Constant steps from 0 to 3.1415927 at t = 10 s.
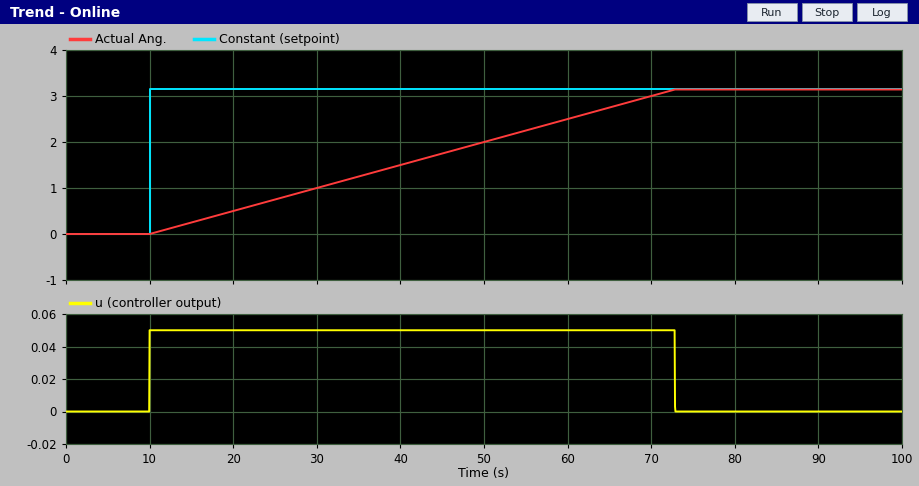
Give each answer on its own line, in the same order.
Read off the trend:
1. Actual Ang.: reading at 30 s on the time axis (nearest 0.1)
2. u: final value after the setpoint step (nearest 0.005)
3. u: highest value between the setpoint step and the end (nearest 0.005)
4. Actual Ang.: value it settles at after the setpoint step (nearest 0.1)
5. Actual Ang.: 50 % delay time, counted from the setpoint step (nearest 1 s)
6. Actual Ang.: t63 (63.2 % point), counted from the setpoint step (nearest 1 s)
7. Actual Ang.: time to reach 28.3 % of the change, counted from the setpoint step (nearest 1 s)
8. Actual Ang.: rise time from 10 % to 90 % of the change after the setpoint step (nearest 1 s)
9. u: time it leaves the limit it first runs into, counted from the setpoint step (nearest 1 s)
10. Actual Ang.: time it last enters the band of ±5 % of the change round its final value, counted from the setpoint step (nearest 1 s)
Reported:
1.0
0.000
0.050
3.1
31 s
40 s
18 s
50 s
63 s
60 s
